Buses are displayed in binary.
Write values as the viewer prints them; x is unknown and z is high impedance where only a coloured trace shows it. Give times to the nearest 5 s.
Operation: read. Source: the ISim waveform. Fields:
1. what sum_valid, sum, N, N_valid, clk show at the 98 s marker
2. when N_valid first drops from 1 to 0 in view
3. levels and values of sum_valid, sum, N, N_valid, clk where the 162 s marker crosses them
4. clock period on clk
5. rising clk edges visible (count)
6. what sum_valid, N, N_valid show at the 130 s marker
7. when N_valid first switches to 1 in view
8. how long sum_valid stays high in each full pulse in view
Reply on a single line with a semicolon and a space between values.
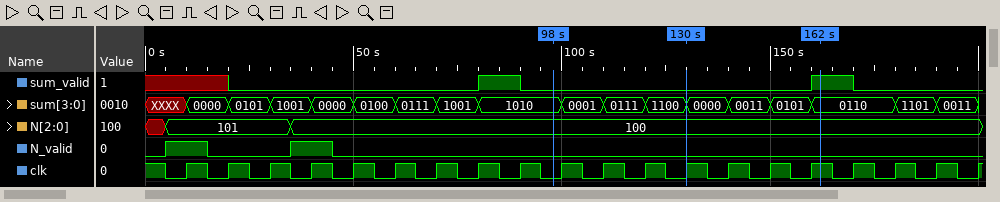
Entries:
sum_valid=0, sum=1010, N=100, N_valid=0, clk=0; 15 s; sum_valid=1, sum=0110, N=100, N_valid=0, clk=1; 10 s; 20; sum_valid=0, N=100, N_valid=0; 5 s; 10 s, 10 s
